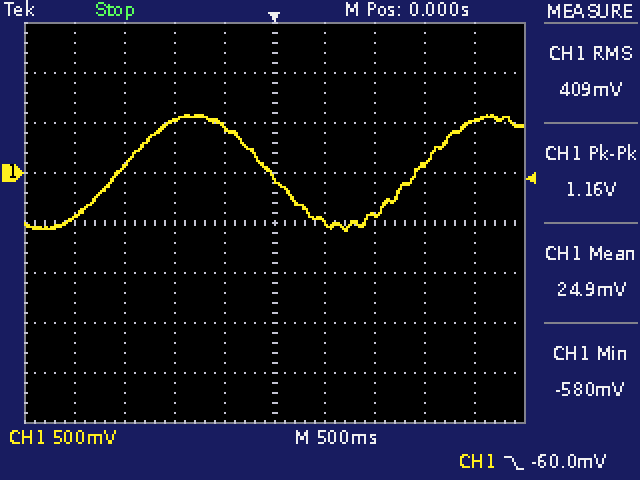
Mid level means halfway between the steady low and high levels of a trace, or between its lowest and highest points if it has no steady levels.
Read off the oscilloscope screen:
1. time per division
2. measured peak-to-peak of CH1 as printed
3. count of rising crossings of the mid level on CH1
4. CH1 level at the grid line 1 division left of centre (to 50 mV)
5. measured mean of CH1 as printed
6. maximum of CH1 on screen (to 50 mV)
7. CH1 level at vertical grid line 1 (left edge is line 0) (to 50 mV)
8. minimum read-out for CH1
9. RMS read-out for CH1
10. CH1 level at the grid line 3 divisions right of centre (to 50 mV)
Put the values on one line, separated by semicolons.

500 ms; 1.16 V; 2; 450 mV; 24.9 mV; 600 mV; -450 mV; -580 mV; 409 mV; 100 mV
